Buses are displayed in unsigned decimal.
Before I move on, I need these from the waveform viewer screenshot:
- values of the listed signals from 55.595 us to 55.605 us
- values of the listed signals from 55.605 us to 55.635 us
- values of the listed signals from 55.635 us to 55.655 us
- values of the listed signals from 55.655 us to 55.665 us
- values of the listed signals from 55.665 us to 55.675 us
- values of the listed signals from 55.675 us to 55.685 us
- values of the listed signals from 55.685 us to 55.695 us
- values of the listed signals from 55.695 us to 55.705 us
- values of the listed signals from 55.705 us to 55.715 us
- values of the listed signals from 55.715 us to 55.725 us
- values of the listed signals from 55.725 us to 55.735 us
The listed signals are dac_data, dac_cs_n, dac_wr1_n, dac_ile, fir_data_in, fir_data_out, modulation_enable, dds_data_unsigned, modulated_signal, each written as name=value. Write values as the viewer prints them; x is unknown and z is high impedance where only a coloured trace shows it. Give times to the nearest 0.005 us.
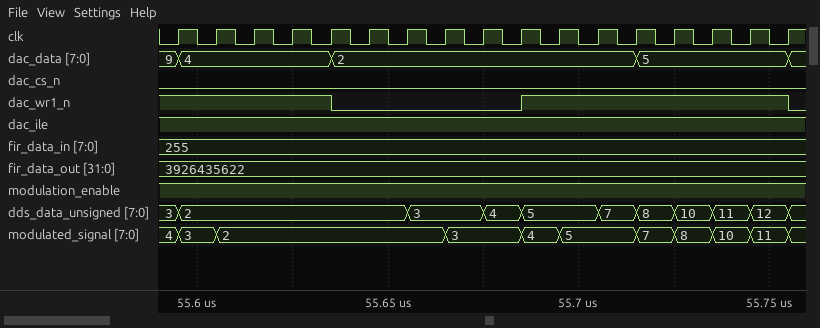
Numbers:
dac_data=4, dac_cs_n=0, dac_wr1_n=1, dac_ile=1, fir_data_in=255, fir_data_out=3926435622, modulation_enable=1, dds_data_unsigned=2, modulated_signal=3
dac_data=4, dac_cs_n=0, dac_wr1_n=1, dac_ile=1, fir_data_in=255, fir_data_out=3926435622, modulation_enable=1, dds_data_unsigned=2, modulated_signal=2
dac_data=2, dac_cs_n=0, dac_wr1_n=0, dac_ile=1, fir_data_in=255, fir_data_out=3926435622, modulation_enable=1, dds_data_unsigned=2, modulated_signal=2
dac_data=2, dac_cs_n=0, dac_wr1_n=0, dac_ile=1, fir_data_in=255, fir_data_out=3926435622, modulation_enable=1, dds_data_unsigned=3, modulated_signal=2
dac_data=2, dac_cs_n=0, dac_wr1_n=0, dac_ile=1, fir_data_in=255, fir_data_out=3926435622, modulation_enable=1, dds_data_unsigned=3, modulated_signal=3
dac_data=2, dac_cs_n=0, dac_wr1_n=0, dac_ile=1, fir_data_in=255, fir_data_out=3926435622, modulation_enable=1, dds_data_unsigned=4, modulated_signal=3
dac_data=2, dac_cs_n=0, dac_wr1_n=1, dac_ile=1, fir_data_in=255, fir_data_out=3926435622, modulation_enable=1, dds_data_unsigned=5, modulated_signal=4
dac_data=2, dac_cs_n=0, dac_wr1_n=1, dac_ile=1, fir_data_in=255, fir_data_out=3926435622, modulation_enable=1, dds_data_unsigned=5, modulated_signal=5
dac_data=2, dac_cs_n=0, dac_wr1_n=1, dac_ile=1, fir_data_in=255, fir_data_out=3926435622, modulation_enable=1, dds_data_unsigned=7, modulated_signal=5
dac_data=5, dac_cs_n=0, dac_wr1_n=1, dac_ile=1, fir_data_in=255, fir_data_out=3926435622, modulation_enable=1, dds_data_unsigned=8, modulated_signal=7
dac_data=5, dac_cs_n=0, dac_wr1_n=1, dac_ile=1, fir_data_in=255, fir_data_out=3926435622, modulation_enable=1, dds_data_unsigned=10, modulated_signal=8
